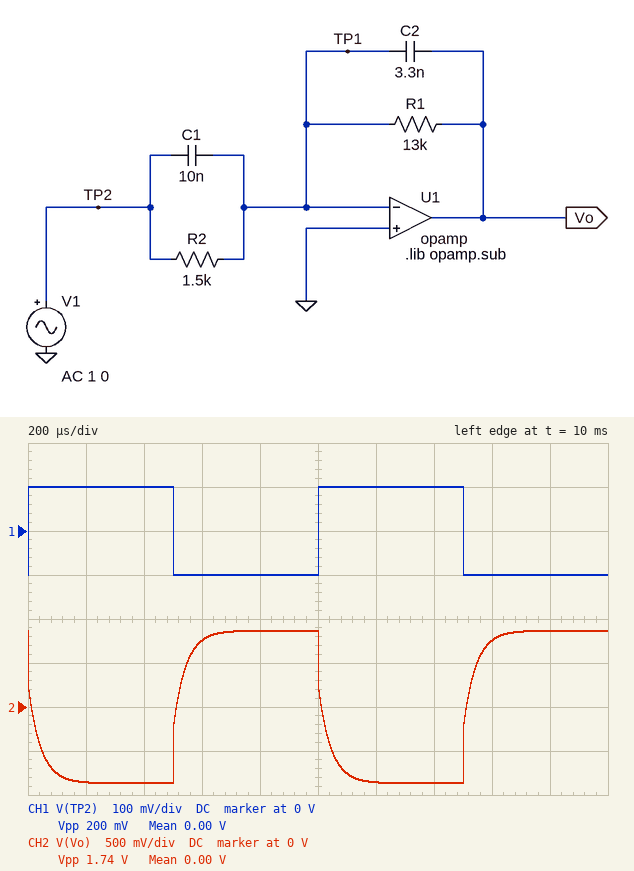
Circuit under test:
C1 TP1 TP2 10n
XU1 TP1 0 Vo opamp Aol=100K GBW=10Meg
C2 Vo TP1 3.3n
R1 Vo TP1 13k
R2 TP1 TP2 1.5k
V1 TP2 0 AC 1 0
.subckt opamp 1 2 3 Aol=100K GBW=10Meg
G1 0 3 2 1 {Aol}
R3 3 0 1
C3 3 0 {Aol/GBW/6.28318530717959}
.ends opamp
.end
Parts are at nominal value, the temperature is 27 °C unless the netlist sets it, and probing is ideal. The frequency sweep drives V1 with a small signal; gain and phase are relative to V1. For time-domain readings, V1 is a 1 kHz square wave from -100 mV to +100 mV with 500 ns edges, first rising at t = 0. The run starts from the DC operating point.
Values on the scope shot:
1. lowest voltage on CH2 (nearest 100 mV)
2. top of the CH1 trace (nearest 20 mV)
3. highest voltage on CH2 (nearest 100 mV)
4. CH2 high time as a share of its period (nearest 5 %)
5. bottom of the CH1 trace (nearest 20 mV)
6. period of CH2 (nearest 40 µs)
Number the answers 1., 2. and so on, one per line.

1. -900 mV
2. 100 mV
3. 900 mV
4. 50 %
5. -100 mV
6. 1.00 ms
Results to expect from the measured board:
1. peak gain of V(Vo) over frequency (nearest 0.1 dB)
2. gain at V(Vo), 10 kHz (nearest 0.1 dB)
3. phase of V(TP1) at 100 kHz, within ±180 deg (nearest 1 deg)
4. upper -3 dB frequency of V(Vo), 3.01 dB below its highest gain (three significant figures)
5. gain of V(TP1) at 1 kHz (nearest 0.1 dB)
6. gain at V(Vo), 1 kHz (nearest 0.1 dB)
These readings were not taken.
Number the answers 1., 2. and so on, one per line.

1. 18.8 dB
2. 12.3 dB
3. 84 deg
4. 4.26 kHz
5. -61.5 dB
6. 18.5 dB
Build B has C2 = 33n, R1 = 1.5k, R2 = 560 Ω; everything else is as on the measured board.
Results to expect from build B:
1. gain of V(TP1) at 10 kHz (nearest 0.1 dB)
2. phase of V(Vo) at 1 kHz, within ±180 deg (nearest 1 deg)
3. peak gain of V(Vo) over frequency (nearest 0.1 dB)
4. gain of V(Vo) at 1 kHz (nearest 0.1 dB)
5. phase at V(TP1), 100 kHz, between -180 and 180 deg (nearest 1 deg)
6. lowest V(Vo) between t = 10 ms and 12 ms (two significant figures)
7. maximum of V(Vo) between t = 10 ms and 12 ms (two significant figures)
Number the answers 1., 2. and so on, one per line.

1. -61.2 dB
2. 165 deg
3. 8.6 dB
4. 8.2 dB
5. 75 deg
6. -270 mV
7. 270 mV
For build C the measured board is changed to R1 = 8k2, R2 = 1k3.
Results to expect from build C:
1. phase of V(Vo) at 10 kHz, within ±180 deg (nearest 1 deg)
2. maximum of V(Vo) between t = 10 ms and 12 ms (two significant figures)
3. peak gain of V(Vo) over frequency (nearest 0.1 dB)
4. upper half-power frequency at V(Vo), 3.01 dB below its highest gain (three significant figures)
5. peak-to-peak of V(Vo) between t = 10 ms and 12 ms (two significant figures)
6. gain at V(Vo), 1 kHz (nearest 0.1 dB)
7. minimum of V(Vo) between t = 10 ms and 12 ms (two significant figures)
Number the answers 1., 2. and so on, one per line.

1. 159 deg
2. 630 mV
3. 16.0 dB
4. 7.99 kHz
5. 1.3 V
6. 15.9 dB
7. -630 mV
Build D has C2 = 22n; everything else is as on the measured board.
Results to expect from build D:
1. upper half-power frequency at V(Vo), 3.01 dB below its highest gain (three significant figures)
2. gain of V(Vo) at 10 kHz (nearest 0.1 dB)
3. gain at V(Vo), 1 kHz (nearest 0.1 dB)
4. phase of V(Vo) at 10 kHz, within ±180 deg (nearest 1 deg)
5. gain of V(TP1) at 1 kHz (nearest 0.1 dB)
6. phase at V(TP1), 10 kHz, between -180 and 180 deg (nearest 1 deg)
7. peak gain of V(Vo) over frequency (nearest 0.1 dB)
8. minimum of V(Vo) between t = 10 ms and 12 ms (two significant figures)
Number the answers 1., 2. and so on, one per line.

1. 558 Hz
2. -3.6 dB
3. 12.5 dB
4. 136 deg
5. -67.4 dB
6. 46 deg
7. 18.8 dB
8. -620 mV
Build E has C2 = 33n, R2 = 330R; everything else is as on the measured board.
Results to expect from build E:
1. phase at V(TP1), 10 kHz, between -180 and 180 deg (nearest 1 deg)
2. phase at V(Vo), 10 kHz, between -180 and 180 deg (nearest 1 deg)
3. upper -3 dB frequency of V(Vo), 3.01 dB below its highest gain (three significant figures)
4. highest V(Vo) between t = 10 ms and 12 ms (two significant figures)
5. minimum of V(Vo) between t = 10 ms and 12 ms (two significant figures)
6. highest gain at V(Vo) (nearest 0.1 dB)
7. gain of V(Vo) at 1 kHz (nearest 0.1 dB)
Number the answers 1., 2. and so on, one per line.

1. 13 deg
2. 104 deg
3. 371 Hz
4. 2.1 V
5. -2.1 V
6. 31.9 dB
7. 22.7 dB
